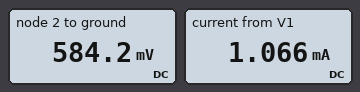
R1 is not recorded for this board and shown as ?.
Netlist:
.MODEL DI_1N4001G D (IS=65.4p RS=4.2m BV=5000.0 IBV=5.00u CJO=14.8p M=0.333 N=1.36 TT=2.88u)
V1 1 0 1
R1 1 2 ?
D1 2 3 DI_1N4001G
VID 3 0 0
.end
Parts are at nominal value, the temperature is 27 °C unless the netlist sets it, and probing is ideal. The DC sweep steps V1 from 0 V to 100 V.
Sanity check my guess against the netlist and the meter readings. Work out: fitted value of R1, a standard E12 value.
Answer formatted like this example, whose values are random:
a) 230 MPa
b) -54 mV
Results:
a) 390 Ω
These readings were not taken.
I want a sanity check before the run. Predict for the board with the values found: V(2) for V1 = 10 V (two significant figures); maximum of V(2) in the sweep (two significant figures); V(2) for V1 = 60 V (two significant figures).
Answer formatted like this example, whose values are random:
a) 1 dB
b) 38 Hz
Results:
a) 690 mV
b) 780 mV
c) 760 mV
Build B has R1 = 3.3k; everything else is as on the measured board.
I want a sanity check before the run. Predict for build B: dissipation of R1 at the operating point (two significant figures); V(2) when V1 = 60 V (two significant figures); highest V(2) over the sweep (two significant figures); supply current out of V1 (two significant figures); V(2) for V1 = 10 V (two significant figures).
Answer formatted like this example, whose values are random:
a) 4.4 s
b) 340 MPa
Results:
a) 71 µW
b) 680 mV
c) 700 mV
d) 150 µA
e) 620 mV
